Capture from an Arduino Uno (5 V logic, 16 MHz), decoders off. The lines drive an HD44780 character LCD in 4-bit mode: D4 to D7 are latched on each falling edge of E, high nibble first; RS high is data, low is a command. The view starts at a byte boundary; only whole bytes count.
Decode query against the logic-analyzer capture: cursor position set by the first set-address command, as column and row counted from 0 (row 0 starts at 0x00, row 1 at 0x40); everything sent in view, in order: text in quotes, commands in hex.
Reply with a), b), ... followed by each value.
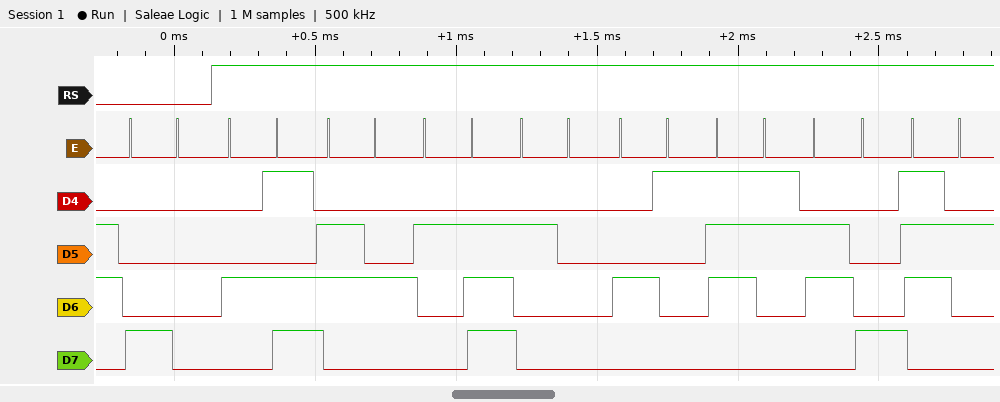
a) column 0, row 0
b) 0x80 "Md. Ashr"
